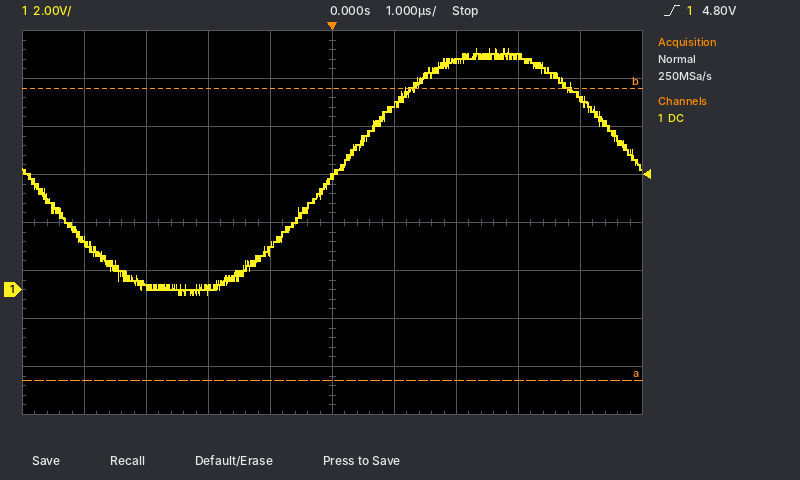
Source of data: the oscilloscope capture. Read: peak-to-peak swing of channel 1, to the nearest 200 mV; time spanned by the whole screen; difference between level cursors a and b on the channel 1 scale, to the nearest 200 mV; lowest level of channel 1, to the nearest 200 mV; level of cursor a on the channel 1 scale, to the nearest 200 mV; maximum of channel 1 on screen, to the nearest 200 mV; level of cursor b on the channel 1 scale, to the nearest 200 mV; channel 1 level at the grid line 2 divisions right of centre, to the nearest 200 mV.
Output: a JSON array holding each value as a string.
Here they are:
["10.2 V", "10 µs", "12.2 V", "-200 mV", "-3.8 V", "10.0 V", "8.4 V", "9.6 V"]
